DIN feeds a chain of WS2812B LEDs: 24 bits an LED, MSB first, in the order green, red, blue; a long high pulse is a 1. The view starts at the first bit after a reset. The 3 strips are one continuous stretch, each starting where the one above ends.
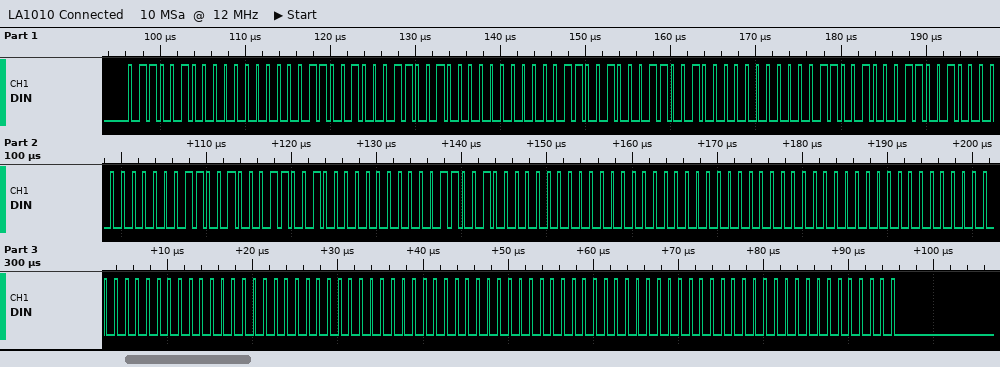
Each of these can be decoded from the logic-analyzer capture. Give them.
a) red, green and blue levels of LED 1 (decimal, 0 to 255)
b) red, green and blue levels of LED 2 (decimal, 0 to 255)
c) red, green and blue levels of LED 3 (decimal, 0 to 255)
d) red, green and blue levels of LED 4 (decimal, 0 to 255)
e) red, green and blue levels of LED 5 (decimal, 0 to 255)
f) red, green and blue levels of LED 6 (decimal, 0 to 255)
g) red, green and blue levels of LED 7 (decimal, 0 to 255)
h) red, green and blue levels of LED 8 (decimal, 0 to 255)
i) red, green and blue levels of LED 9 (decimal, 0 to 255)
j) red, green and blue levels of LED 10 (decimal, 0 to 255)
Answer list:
0, 100, 100
0, 100, 100
0, 100, 100
0, 100, 100
0, 100, 100
0, 0, 0
0, 0, 0
0, 0, 0
0, 0, 0
0, 0, 0
